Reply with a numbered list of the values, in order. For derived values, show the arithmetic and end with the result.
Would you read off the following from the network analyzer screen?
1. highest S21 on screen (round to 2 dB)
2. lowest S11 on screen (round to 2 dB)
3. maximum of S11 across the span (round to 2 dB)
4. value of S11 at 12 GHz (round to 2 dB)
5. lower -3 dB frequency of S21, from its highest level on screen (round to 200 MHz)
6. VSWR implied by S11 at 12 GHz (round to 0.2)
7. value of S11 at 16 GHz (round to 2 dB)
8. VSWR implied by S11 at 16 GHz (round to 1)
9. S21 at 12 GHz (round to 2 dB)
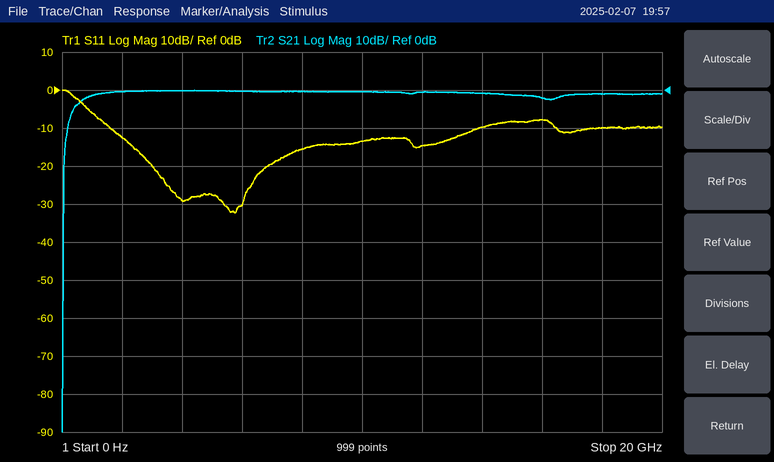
1. 0 dB
2. -32 dB
3. 0 dB
4. -14 dB
5. 600 MHz
6. |Γ| = 10^(-14/20) = 0.1995; VSWR = (1 + 0.1995)/(1 − 0.1995) ≈ 1.50, so 1.4 to the nearest 0.2
7. -8 dB
8. |Γ| = 10^(-8/20) = 0.3981; VSWR = (1 + 0.3981)/(1 − 0.3981) ≈ 2
9. 0 dB
